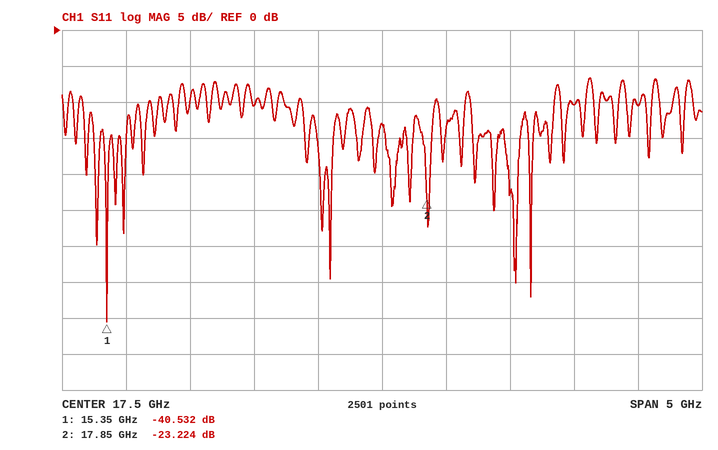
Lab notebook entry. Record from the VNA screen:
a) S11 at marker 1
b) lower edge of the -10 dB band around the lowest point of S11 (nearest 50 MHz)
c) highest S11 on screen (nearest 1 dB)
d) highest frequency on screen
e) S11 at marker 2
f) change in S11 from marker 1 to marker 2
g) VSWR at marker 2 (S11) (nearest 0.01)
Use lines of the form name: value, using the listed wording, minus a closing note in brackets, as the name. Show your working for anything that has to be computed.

S11 at marker 1: -40.532 dB
lower edge of the -10 dB band around the lowest point of S11: 15.15 GHz
highest S11 on screen: -7 dB
highest frequency on screen: 20 GHz
S11 at marker 2: -23.224 dB
change in S11 from marker 1 to marker 2: -23.224 − (-40.532) = 17.308 dB
VSWR at marker 2 (S11): (1 + 0.0690)/(1 − 0.0690) ≈ 1.15
